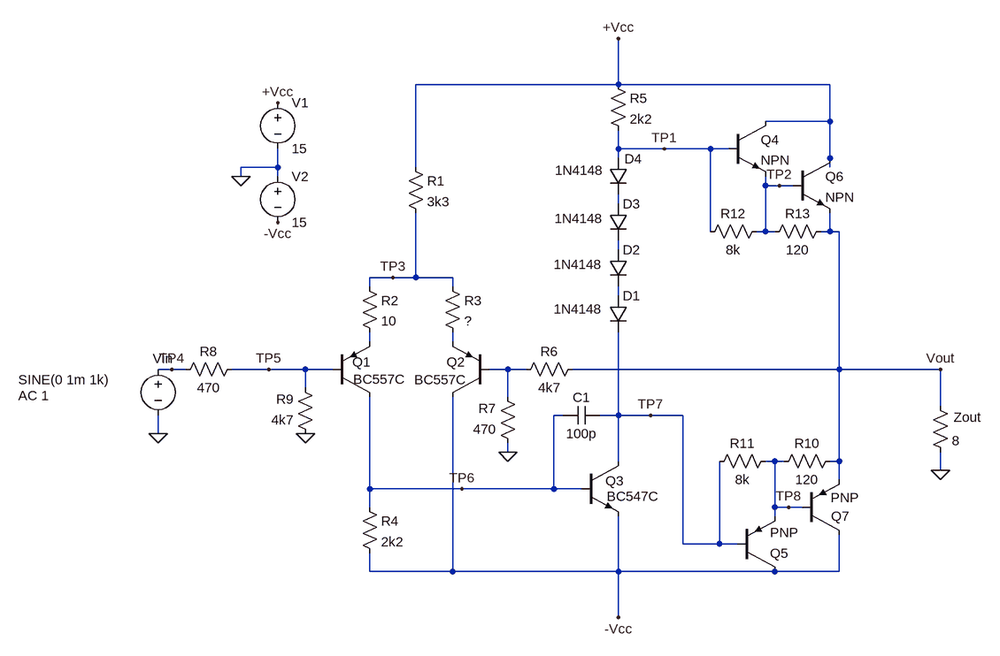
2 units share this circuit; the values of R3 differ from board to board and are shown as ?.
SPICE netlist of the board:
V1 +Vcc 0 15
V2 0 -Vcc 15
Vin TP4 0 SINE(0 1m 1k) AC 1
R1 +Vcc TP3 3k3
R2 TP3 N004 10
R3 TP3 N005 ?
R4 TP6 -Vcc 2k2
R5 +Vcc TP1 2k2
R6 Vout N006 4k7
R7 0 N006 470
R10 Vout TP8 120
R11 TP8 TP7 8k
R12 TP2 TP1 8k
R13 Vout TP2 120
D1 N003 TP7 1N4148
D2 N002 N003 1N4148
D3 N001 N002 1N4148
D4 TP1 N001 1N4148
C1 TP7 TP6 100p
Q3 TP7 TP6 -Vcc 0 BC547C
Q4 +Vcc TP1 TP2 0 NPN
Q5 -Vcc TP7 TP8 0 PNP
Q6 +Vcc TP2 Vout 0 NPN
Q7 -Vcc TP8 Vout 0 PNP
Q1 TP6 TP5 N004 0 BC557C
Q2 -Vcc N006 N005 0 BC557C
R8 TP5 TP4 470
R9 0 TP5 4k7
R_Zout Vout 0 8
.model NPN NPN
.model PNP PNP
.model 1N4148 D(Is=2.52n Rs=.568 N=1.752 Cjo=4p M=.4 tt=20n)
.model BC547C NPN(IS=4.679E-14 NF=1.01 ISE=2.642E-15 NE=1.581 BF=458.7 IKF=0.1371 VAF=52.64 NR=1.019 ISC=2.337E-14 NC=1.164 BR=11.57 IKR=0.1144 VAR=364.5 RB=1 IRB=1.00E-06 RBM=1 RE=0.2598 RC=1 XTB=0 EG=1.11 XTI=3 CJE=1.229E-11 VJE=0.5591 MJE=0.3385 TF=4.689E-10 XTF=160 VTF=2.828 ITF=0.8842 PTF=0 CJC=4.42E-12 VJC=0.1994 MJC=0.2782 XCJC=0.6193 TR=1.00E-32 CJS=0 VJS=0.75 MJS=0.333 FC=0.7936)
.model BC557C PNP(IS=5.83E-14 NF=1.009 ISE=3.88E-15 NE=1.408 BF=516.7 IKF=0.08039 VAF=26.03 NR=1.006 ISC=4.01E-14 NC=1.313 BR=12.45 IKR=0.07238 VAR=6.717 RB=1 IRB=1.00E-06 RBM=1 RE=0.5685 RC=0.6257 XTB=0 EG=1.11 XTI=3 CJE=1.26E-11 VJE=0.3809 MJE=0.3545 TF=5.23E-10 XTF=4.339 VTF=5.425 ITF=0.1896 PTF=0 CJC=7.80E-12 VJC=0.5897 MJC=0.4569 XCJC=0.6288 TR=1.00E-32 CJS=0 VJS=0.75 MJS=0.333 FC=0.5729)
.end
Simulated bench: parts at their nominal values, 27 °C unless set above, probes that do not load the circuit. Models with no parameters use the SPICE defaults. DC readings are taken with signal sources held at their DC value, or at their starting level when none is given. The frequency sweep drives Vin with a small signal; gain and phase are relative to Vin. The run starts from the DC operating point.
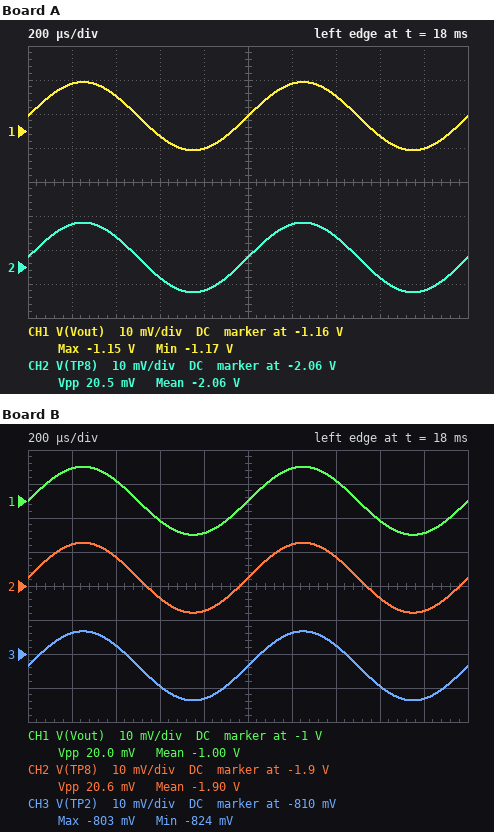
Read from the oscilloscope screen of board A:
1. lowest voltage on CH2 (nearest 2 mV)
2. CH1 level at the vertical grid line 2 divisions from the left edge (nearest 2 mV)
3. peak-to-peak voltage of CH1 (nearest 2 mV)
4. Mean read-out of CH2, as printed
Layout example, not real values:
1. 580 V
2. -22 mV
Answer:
1. -2.068 V
2. -1.150 V
3. 20 mV
4. -2.06 V
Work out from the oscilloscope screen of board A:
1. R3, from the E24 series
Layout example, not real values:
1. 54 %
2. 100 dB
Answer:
1. 9.1 Ω
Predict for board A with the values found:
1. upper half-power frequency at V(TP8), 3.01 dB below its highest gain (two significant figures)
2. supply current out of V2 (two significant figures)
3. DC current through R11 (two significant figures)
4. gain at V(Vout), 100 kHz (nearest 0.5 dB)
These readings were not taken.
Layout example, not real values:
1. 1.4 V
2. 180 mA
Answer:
1. 1.4 MHz
2. 160 mA
3. 100 µA
4. 20.0 dB
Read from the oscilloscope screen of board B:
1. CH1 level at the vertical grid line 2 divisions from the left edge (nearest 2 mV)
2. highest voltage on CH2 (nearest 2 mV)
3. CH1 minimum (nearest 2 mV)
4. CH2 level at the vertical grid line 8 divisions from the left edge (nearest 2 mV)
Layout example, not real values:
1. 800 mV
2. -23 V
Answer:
1. -994 mV
2. -1.888 V
3. -1.010 V
4. -1.904 V
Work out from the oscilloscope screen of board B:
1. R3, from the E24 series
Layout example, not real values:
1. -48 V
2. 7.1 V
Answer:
1. 5.6 Ω
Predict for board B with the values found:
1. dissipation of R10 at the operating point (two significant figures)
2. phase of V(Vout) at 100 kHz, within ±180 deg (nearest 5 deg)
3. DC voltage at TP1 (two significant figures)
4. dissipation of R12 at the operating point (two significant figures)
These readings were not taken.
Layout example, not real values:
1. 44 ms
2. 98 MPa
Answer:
1. 6.7 mW
2. -5 deg
3. -30 mV
4. 77 µW
